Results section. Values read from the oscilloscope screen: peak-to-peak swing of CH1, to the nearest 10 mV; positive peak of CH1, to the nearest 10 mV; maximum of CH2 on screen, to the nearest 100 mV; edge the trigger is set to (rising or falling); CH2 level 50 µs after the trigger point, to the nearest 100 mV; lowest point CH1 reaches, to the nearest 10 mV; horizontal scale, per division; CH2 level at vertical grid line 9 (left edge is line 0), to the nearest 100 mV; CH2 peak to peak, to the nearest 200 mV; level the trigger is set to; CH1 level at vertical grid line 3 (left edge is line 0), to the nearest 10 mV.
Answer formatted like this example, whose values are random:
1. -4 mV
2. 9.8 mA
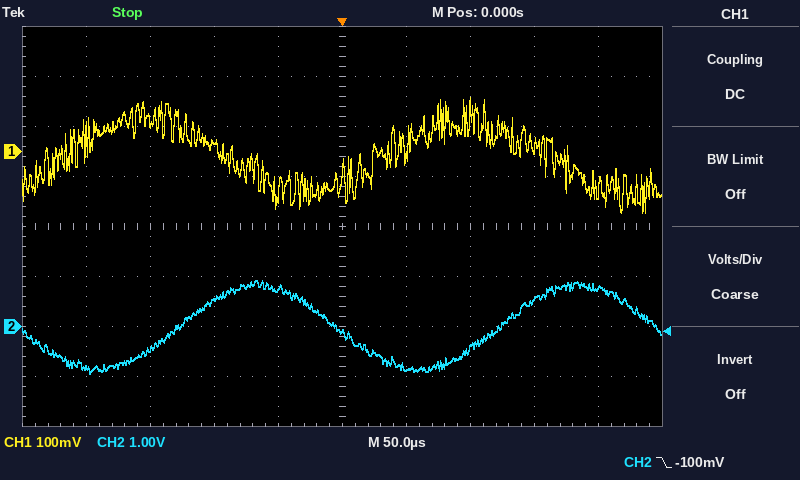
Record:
1. 230 mV
2. 110 mV
3. 900 mV
4. falling
5. -800 mV
6. -120 mV
7. 50 µs
8. 800 mV
9. 1.8 V
10. -100 mV
11. 20 mV
